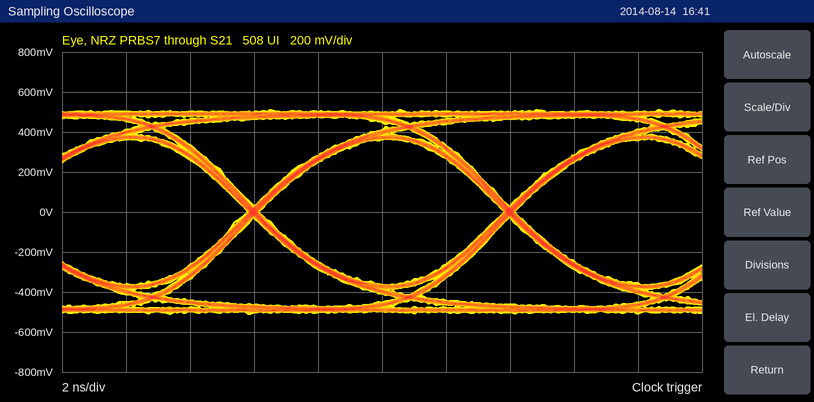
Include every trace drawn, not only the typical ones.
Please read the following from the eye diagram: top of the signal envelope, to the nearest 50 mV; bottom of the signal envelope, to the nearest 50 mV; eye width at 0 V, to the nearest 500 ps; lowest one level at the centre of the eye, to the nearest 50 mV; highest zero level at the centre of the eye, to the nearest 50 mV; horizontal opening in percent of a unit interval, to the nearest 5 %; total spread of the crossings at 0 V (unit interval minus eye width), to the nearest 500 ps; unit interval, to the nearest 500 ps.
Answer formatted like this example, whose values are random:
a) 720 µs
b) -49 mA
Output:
a) 500 mV
b) -500 mV
c) 7.5 ns
d) 350 mV
e) -350 mV
f) 95 %
g) 500 ps
h) 8.0 ns
